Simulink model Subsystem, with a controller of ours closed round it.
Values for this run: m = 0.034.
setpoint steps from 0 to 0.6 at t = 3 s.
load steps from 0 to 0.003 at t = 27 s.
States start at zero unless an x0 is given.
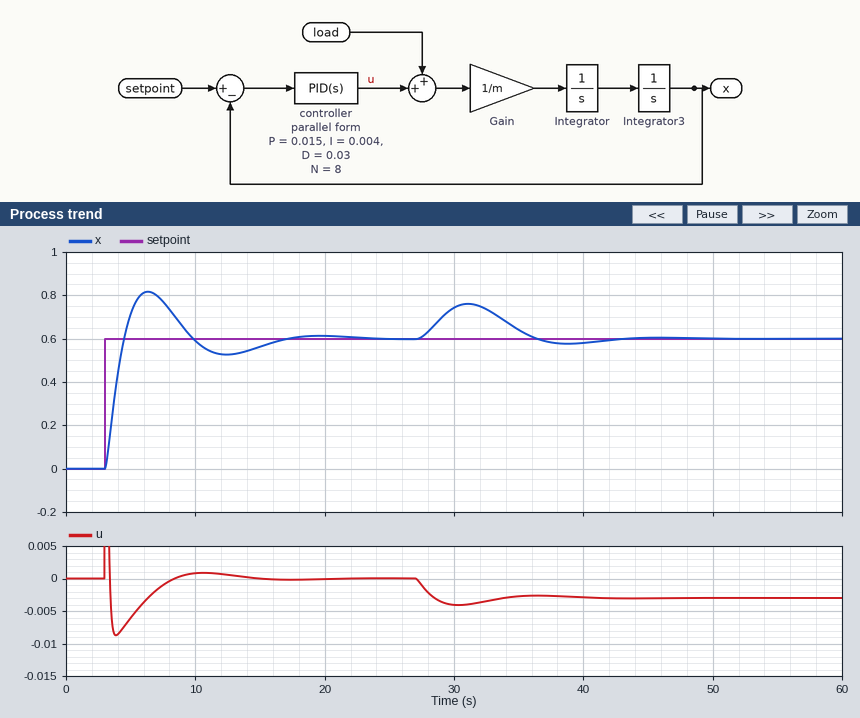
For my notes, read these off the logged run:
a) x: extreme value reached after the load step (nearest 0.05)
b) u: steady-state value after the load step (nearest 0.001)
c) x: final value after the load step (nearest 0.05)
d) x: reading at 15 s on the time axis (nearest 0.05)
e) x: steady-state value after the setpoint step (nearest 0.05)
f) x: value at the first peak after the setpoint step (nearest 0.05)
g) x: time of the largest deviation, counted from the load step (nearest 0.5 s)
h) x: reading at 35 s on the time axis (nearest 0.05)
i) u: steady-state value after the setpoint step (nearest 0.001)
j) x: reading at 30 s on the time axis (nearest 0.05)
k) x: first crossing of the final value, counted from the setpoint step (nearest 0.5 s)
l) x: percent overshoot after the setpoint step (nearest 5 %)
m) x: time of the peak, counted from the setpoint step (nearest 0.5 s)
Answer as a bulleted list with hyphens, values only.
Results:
- 0.75
- -0.003
- 0.60
- 0.55
- 0.60
- 0.80
- 4.0 s
- 0.65
- 0.000
- 0.75
- 1.5 s
- 35 %
- 3.5 s
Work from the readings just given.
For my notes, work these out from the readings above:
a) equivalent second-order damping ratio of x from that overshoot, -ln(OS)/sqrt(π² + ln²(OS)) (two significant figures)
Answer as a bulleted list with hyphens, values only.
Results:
- 0.32
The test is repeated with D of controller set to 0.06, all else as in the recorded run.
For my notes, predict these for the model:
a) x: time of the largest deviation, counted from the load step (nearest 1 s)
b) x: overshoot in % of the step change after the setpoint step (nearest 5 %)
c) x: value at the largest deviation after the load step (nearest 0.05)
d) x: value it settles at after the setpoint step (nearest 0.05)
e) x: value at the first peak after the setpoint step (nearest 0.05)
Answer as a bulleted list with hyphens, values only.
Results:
- 5 s
- 15 %
- 0.70
- 0.60
- 0.70
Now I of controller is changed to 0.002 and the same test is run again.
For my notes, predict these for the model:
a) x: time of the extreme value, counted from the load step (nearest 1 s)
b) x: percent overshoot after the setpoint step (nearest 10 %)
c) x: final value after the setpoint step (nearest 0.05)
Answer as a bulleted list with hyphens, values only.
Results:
- 5 s
- 30 %
- 0.60
